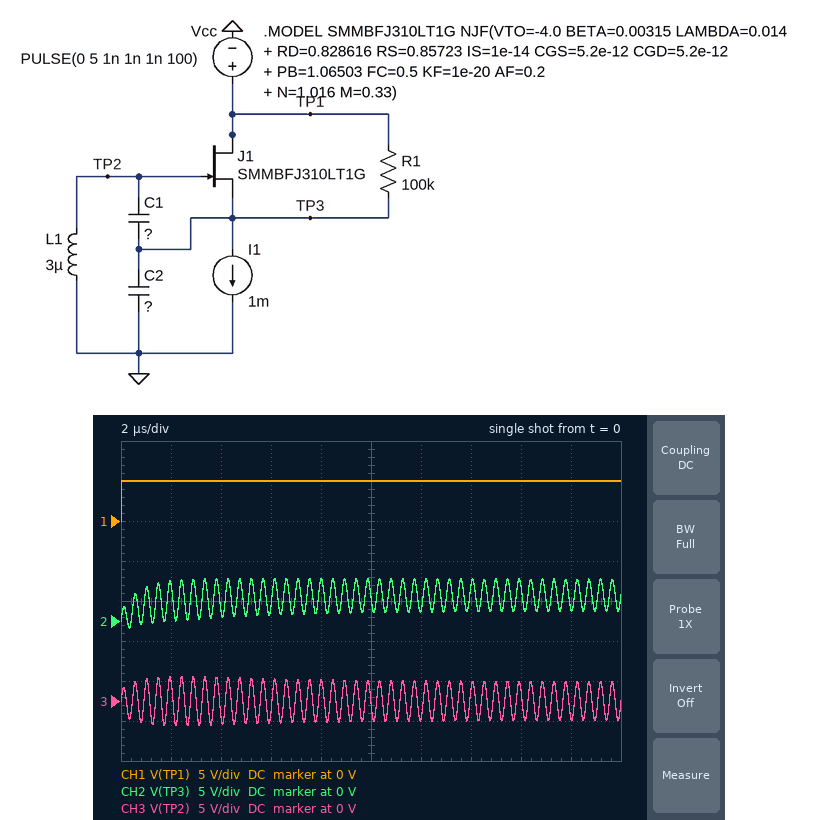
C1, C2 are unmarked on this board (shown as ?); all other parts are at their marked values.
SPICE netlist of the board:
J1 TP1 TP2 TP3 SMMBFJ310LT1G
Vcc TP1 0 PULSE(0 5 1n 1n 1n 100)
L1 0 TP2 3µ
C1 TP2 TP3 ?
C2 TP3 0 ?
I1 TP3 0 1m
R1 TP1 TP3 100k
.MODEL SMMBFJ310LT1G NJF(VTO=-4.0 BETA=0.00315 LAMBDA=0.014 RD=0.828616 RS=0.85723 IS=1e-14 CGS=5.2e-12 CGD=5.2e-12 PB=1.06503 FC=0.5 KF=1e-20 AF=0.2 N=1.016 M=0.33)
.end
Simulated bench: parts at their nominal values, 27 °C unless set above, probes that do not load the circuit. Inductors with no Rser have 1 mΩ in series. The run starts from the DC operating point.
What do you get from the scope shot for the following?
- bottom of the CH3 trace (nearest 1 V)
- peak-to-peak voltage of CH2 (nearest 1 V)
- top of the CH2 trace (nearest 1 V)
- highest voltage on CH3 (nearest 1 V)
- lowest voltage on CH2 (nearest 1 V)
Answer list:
-3 V
6 V
5 V
3 V
-1 V
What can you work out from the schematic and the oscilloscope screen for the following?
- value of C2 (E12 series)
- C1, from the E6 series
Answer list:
2.2 nF
10 nF
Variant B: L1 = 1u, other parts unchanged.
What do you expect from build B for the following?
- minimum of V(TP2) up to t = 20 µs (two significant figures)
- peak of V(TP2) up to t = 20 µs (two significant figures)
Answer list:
-2.6 V
2.6 V
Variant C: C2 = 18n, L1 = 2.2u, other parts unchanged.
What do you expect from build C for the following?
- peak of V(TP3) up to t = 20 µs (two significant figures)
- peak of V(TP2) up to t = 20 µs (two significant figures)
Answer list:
4.7 V
2.7 V
